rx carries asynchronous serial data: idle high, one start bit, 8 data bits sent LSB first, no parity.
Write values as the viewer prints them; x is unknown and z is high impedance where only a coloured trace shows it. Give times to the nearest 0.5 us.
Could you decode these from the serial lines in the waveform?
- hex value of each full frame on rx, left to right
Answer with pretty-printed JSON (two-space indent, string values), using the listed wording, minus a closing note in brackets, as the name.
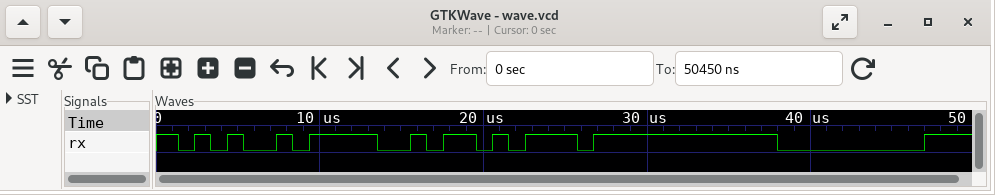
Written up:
{
  "hex value of each full frame on rx, left to right": "A5, 5A, FF, 00"
}
